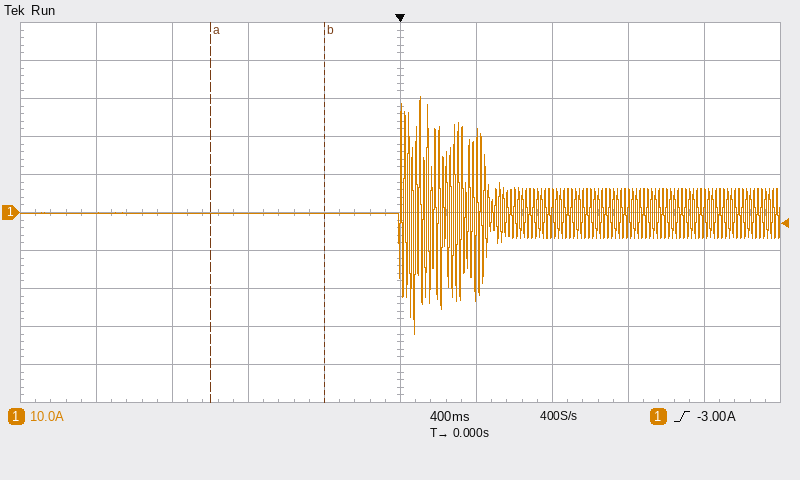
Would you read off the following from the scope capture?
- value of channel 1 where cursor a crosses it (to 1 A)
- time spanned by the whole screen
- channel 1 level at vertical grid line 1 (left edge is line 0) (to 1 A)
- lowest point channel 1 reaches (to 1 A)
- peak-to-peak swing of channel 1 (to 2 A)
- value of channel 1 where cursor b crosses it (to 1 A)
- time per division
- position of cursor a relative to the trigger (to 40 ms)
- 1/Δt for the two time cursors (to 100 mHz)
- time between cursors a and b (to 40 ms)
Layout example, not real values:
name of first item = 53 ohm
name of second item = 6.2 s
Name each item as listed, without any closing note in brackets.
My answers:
value of channel 1 where cursor a crosses it = 0 A
time spanned by the whole screen = 4 s
channel 1 level at vertical grid line 1 (left edge is line 0) = 0 A
lowest point channel 1 reaches = -32 A
peak-to-peak swing of channel 1 = 62 A
value of channel 1 where cursor b crosses it = 0 A
time per division = 400 ms
position of cursor a relative to the trigger = -1.00 s
1/Δt for the two time cursors = 1.7 Hz
time between cursors a and b = 600 ms
